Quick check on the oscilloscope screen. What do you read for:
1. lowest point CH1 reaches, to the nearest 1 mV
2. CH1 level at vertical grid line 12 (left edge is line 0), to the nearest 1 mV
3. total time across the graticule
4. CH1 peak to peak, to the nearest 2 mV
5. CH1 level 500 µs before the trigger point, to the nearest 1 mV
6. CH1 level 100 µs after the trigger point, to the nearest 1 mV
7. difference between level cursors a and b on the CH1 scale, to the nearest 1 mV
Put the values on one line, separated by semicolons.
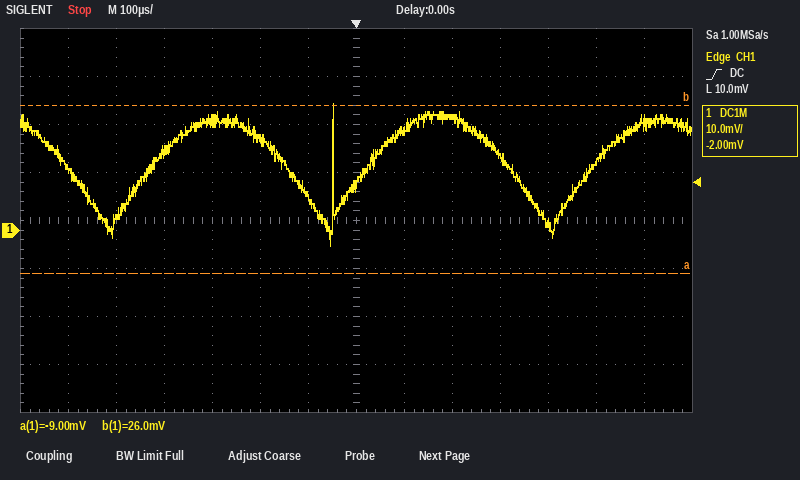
-3 mV; 14 mV; 1.4 ms; 30 mV; 2 mV; 21 mV; 35 mV
